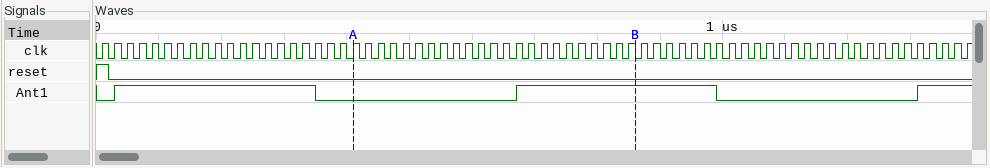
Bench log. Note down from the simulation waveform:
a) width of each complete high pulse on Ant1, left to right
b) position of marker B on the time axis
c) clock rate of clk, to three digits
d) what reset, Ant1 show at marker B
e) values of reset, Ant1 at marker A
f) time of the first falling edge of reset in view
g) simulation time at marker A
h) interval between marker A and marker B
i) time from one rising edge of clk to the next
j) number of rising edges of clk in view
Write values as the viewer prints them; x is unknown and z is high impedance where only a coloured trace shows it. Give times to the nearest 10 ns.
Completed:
320 ns, 320 ns
860 ns
50.0 MHz
reset=0, Ant1=1
reset=0, Ant1=0
20 ns
410 ns
450 ns
20 ns
70
